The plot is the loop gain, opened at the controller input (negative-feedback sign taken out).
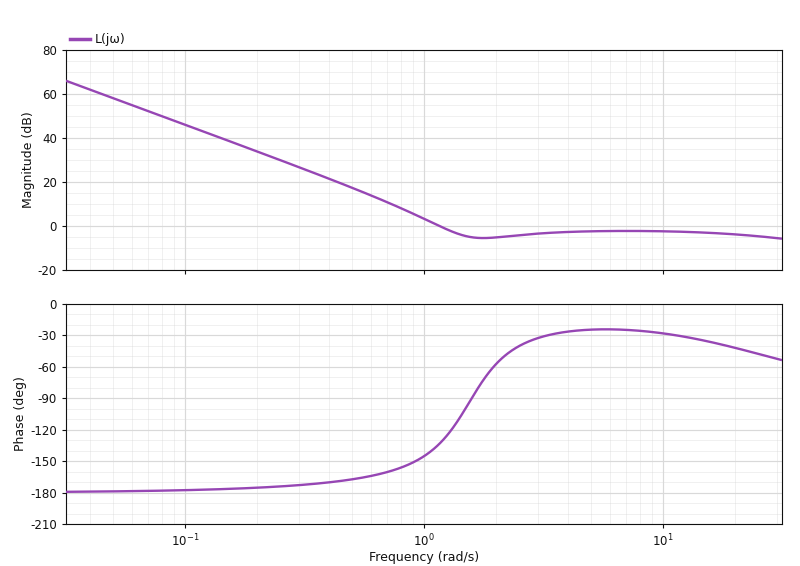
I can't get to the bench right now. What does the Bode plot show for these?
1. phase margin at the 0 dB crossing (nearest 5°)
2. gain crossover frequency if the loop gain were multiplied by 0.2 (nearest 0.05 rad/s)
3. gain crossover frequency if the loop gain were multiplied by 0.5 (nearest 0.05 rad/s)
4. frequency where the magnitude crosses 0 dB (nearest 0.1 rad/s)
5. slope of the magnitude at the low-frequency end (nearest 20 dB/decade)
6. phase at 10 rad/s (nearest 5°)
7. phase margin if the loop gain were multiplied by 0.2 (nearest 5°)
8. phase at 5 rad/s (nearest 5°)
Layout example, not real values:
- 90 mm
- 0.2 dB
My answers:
- 45°
- 0.60 rad/s
- 0.90 rad/s
- 1.2 rad/s
- -40 dB/decade
- -30°
- 15°
- -25°
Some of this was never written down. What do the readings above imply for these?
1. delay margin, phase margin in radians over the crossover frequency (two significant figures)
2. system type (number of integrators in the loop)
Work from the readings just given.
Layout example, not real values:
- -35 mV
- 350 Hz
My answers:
- 0.65 s
- 2
